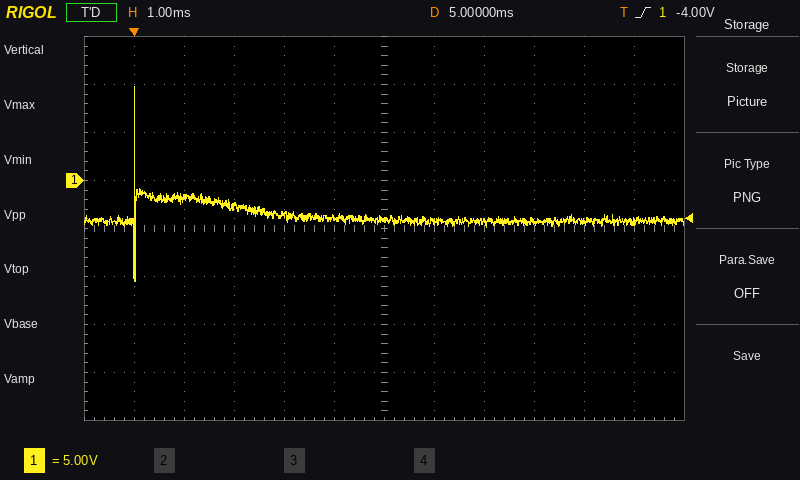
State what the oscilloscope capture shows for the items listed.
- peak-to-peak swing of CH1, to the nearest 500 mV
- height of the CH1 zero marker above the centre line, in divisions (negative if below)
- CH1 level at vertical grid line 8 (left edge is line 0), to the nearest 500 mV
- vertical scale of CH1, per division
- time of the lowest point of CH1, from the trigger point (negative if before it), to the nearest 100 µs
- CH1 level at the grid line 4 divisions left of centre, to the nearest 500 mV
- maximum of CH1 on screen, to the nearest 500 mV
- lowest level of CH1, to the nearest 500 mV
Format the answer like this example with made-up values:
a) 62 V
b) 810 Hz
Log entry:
a) 20.5 V
b) +1.0 div
c) -4.5 V
d) 5 V
e) 0.0 ms
f) -2.0 V
g) 10.0 V
h) -10.5 V
